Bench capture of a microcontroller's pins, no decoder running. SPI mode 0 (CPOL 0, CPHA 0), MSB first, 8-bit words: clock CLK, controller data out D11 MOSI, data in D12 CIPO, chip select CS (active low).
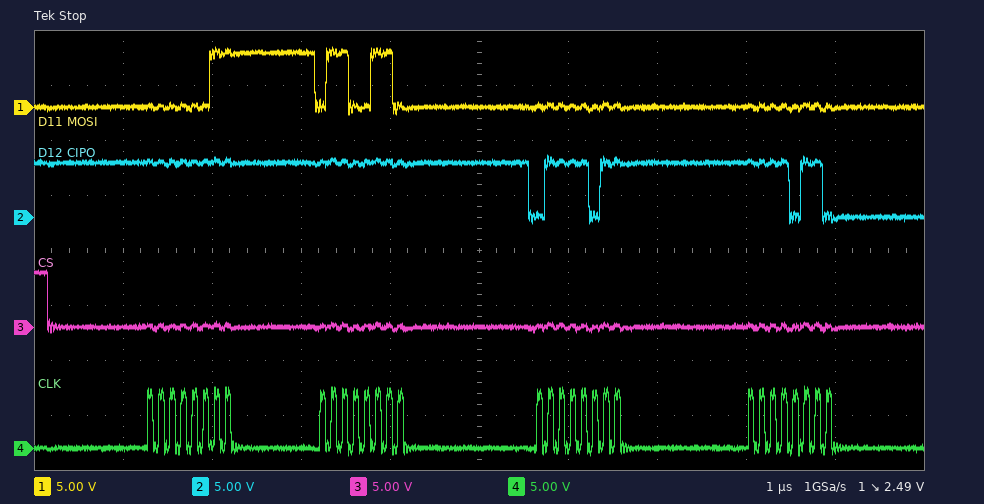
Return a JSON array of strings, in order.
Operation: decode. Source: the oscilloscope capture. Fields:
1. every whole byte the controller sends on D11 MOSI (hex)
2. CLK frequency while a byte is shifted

["03 66 00 00", "8 MHz"]
